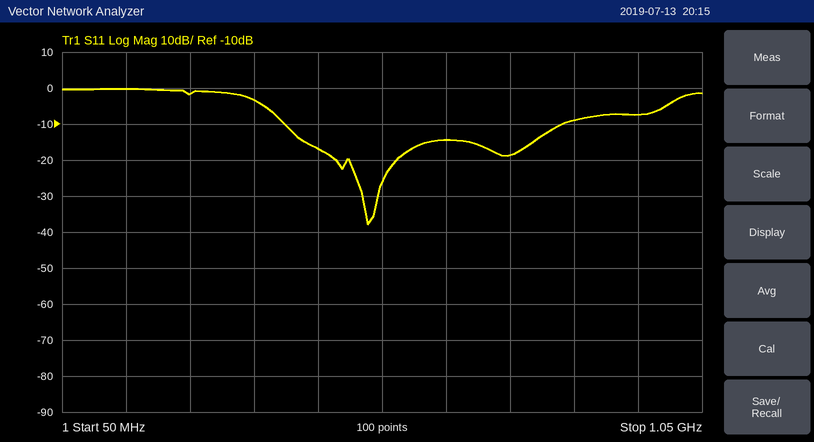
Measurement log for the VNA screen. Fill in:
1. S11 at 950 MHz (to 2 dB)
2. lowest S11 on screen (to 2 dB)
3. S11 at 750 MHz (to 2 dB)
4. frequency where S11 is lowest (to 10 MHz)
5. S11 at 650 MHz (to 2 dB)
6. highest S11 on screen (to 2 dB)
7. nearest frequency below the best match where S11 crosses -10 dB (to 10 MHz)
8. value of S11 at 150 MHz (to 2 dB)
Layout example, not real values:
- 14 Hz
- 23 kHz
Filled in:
- -8 dB
- -38 dB
- -18 dB
- 530 MHz
- -14 dB
- 0 dB
- 400 MHz
- 0 dB
